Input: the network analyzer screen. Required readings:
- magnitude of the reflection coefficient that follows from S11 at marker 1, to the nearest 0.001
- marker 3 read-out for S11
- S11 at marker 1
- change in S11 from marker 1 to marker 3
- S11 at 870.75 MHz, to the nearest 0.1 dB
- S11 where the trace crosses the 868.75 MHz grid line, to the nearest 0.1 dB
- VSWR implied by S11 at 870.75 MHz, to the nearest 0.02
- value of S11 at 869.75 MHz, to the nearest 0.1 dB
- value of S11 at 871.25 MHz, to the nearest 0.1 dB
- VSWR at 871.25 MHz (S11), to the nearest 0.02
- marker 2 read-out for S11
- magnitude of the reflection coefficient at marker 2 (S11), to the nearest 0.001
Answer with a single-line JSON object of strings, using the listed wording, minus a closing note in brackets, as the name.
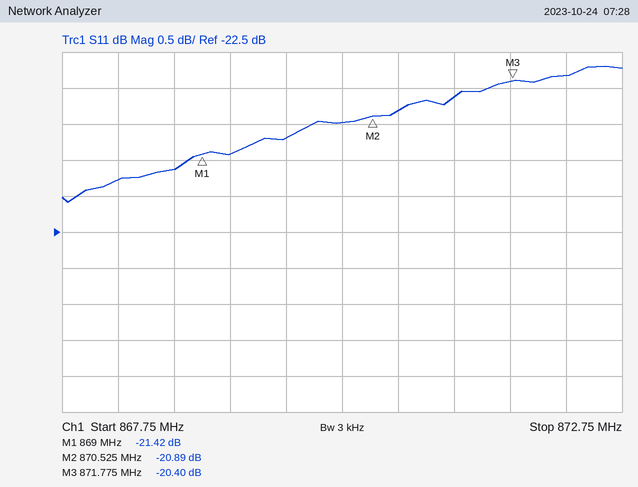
{"magnitude of the reflection coefficient that follows from S11 at marker 1, to the nearest 0.001": "0.085", "marker 3 read-out for S11": "-20.40 dB", "S11 at marker 1": "-21.42 dB", "change in S11 from marker 1 to marker 3": "1.02 dB", "S11 at 870.75 MHz, to the nearest 0.1 dB": "-20.8 dB", "S11 where the trace crosses the 868.75 MHz grid line, to the nearest 0.1 dB": "-21.6 dB", "VSWR implied by S11 at 870.75 MHz, to the nearest 0.02": "1.20", "value of S11 at 869.75 MHz, to the nearest 0.1 dB": "-21.2 dB", "value of S11 at 871.25 MHz, to the nearest 0.1 dB": "-20.6 dB", "VSWR at 871.25 MHz (S11), to the nearest 0.02": "1.20", "marker 2 read-out for S11": "-20.89 dB", "magnitude of the reflection coefficient at marker 2 (S11), to the nearest 0.001": "0.090"}
